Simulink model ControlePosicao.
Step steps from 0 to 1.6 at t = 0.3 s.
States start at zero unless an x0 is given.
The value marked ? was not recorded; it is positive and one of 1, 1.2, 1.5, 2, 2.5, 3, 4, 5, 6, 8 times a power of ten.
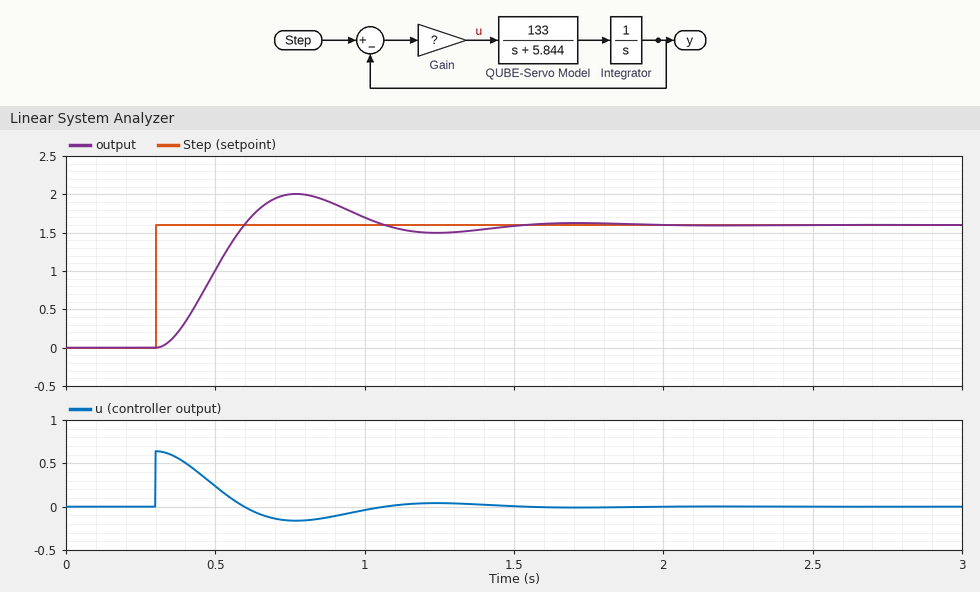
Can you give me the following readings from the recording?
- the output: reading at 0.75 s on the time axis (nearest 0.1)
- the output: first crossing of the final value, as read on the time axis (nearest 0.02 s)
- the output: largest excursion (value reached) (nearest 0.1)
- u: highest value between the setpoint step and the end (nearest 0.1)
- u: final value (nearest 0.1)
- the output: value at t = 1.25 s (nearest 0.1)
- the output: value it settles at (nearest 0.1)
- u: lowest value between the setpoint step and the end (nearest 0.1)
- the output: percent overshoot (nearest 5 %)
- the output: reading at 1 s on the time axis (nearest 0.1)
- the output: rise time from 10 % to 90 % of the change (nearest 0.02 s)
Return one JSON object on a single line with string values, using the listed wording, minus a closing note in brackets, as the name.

{"the output: reading at 0.75 s on the time axis": "2.0", "the output: first crossing of the final value, as read on the time axis": "0.60 s", "the output: largest excursion (value reached)": "2.0", "u: highest value between the setpoint step and the end": "0.6", "u: final value": "0.0", "the output: value at t = 1.25 s": "1.5", "the output: value it settles at": "1.6", "u: lowest value between the setpoint step and the end": "-0.2", "the output: percent overshoot": "25 %", "the output: reading at 1 s on the time axis": "1.7", "the output: rise time from 10 % to 90 % of the change": "0.20 s"}
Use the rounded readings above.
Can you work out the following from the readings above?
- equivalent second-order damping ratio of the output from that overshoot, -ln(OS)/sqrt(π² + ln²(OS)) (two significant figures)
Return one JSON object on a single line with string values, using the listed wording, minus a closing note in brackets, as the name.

{"equivalent second-order damping ratio of the output from that overshoot, -ln(OS)/sqrt(π² + ln²(OS))": "0.40"}
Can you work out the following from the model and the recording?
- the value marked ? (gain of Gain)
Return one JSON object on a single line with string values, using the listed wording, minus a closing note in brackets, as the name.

{"the value marked ?": "0.4"}
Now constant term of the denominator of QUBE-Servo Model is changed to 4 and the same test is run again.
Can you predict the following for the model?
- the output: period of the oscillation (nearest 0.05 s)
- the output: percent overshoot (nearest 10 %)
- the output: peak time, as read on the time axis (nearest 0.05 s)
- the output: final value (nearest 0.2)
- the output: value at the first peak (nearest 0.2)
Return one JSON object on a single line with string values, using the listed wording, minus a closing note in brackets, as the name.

{"the output: period of the oscillation": "0.90 s", "the output: percent overshoot": "40 %", "the output: peak time, as read on the time axis": "0.75 s", "the output: final value": "1.6", "the output: value at the first peak": "2.2"}
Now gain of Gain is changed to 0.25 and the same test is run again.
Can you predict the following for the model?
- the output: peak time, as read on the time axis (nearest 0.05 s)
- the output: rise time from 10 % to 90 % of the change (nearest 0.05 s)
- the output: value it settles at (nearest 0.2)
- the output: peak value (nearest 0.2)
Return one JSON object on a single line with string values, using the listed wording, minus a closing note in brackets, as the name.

{"the output: peak time, as read on the time axis": "0.95 s", "the output: rise time from 10 % to 90 % of the change": "0.30 s", "the output: value it settles at": "1.6", "the output: peak value": "1.8"}
